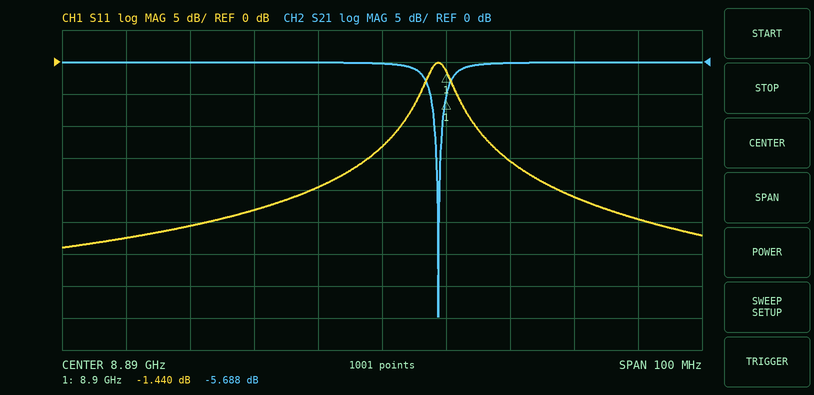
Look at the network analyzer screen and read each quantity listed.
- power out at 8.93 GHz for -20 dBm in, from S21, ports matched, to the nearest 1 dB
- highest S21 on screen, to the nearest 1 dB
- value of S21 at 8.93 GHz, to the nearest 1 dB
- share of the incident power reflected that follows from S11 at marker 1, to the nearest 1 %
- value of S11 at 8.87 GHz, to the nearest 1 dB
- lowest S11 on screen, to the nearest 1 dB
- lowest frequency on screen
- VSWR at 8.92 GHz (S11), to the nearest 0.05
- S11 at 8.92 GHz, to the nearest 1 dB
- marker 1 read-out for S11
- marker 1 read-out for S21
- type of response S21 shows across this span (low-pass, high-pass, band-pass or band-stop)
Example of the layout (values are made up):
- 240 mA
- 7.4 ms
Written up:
- -20 dBm
- 0 dB
- 0 dB
- 72 %
- -23 dB
- -29 dB
- 8.84 GHz
- 1.20
- -21 dB
- -1.440 dB
- -5.688 dB
- band-stop
